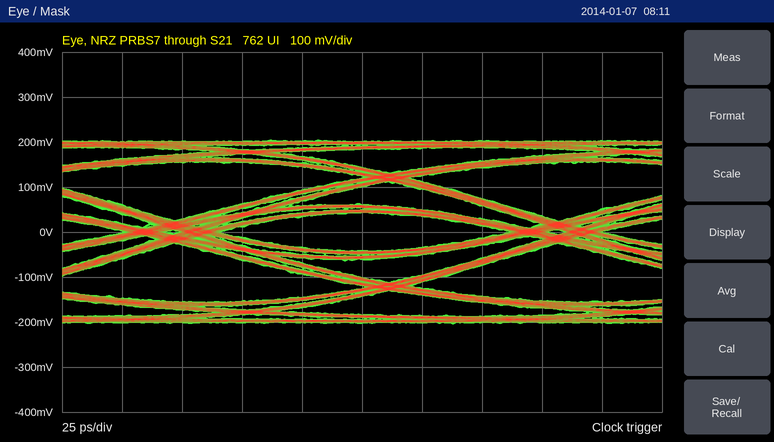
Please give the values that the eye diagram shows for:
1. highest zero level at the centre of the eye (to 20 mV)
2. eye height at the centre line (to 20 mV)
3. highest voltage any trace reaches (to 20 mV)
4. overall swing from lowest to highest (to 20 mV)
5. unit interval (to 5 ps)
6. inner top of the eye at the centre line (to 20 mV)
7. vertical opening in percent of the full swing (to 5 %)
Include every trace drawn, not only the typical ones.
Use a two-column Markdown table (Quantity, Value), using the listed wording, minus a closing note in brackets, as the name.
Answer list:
| Quantity | Value |
|---|---|
| highest zero level at the centre of the eye | -40 mV |
| eye height at the centre line | 80 mV |
| highest voltage any trace reaches | 200 mV |
| overall swing from lowest to highest | 400 mV |
| unit interval | 160 ps |
| inner top of the eye at the centre line | 40 mV |
| vertical opening in percent of the full swing | 20 % |
